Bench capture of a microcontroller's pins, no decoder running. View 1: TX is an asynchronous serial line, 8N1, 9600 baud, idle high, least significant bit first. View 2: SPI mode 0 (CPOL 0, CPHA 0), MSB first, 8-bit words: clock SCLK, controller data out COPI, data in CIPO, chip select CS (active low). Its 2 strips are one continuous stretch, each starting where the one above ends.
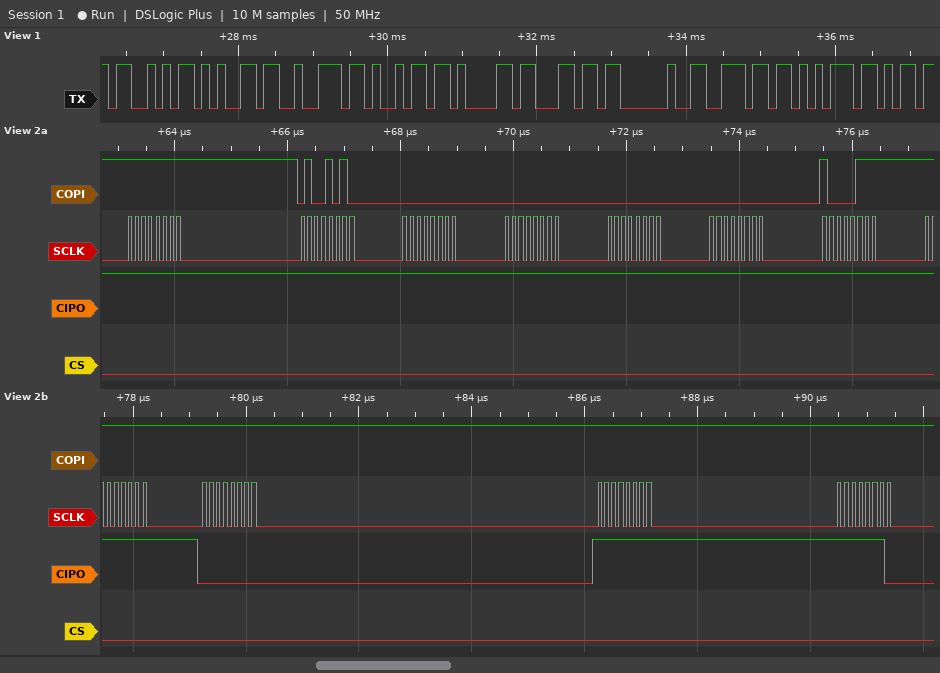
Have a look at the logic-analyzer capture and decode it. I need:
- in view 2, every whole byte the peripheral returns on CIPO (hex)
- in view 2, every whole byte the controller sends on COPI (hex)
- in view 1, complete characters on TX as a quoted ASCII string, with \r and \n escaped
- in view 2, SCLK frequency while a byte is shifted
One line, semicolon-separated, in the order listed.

0xFF 0xFF 0xFF 0xFF 0xFF 0xFF 0xFF 0xFF 0x00 0xFF 0xFE; 0xFF 0x4A 0x00 0x00 0x00 0x00 0x87 0xFF 0xFF 0xFF 0xFF; "Serial nu"; 8 MHz
